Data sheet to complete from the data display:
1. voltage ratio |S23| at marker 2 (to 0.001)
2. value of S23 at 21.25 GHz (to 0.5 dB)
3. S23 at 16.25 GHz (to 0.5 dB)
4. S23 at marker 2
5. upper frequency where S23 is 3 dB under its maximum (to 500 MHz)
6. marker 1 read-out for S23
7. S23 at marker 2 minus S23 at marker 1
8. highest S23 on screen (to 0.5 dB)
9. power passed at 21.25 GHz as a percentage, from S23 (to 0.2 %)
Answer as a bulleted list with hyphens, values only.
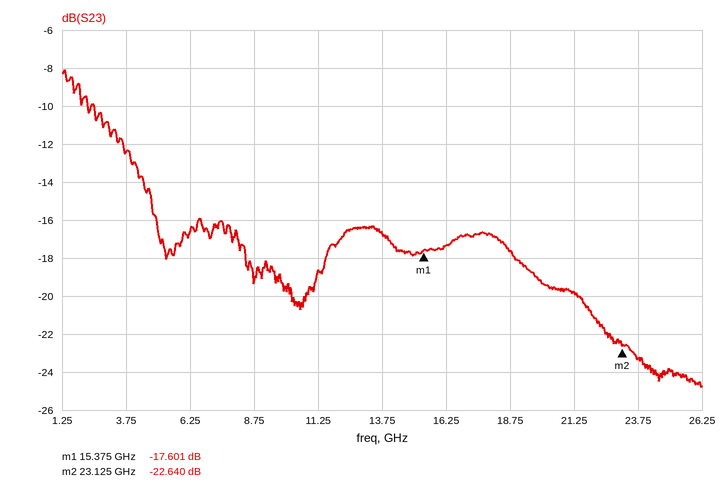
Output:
- 0.074
- -20.0 dB
- -17.5 dB
- -22.640 dB
- 3.0 GHz
- -17.601 dB
- -5.039 dB
- -8.0 dB
- 1.0 %
